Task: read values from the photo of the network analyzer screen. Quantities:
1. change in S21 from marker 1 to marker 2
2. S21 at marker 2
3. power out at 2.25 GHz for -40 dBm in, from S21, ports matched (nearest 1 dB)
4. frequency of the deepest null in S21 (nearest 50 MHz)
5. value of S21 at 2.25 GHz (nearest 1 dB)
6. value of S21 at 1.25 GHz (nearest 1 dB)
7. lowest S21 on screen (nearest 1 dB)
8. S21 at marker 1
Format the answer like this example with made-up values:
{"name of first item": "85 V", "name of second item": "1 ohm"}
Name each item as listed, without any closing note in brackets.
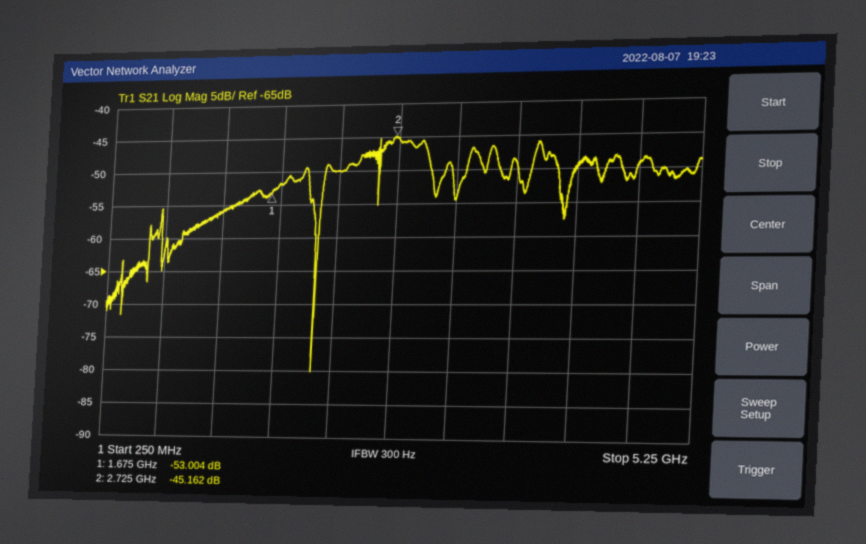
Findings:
{"change in S21 from marker 1 to marker 2": "7.842 dB", "S21 at marker 2": "-45.162 dB", "power out at 2.25 GHz for -40 dBm in, from S21, ports matched": "-90 dBm", "frequency of the deepest null in S21": "2.10 GHz", "value of S21 at 2.25 GHz": "-50 dB", "value of S21 at 1.25 GHz": "-56 dB", "lowest S21 on screen": "-80 dB", "S21 at marker 1": "-53.004 dB"}
